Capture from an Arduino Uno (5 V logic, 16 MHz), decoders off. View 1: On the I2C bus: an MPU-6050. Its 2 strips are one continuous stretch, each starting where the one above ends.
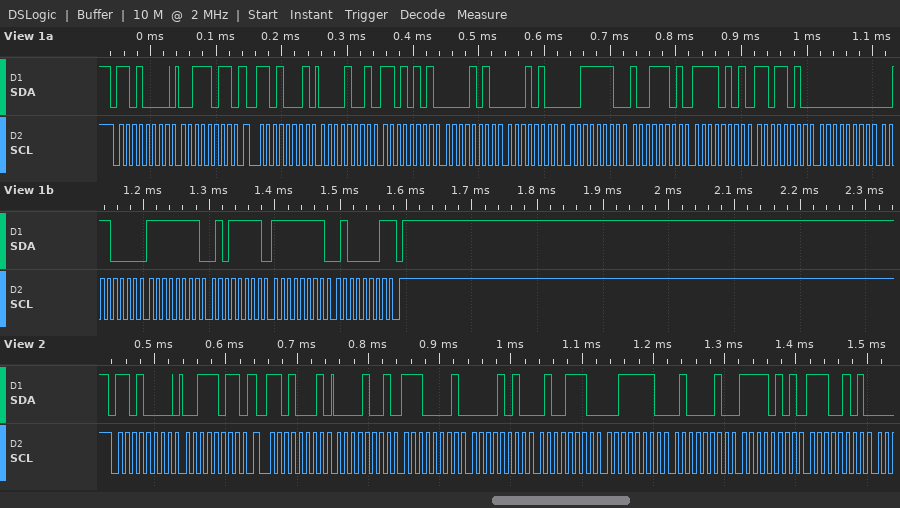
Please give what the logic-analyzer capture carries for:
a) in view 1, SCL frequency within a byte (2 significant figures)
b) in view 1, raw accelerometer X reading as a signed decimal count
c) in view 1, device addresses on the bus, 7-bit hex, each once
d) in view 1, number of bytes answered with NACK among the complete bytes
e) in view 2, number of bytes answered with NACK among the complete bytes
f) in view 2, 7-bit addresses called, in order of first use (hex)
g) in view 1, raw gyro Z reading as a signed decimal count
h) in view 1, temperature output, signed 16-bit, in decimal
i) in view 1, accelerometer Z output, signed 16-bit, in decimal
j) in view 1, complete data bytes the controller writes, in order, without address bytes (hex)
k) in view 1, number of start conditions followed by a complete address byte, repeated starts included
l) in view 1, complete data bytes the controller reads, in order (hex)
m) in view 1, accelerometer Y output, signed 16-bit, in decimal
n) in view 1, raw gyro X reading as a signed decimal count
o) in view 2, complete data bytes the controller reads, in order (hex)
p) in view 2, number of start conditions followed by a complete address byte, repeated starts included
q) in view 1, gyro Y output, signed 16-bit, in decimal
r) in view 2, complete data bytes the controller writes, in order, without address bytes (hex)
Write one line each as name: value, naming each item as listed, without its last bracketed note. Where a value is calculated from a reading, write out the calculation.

in view 1, SCL frequency within a byte: 100 kHz
in view 1, raw accelerometer X reading as a signed decimal count: 0x09D5 = 2517
in view 1, device addresses on the bus, 7-bit hex, each once: 0x68
in view 1, number of bytes answered with NACK among the complete bytes: 1
in view 2, number of bytes answered with NACK among the complete bytes: 0
in view 2, 7-bit addresses called, in order of first use: 0x68
in view 1, raw gyro Z reading as a signed decimal count: 0xFF41 = -191
in view 1, temperature output, signed 16-bit, in decimal: 0xF5DA = -2598
in view 1, accelerometer Z output, signed 16-bit, in decimal: 0x3E9D = 16029
in view 1, complete data bytes the controller writes, in order, without address bytes: 3B
in view 1, number of start conditions followed by a complete address byte, repeated starts included: 2
in view 1, complete data bytes the controller reads, in order: 09 D5 0A 14 3E 9D F5 DA 00 30 FF 5F FF 41
in view 1, accelerometer Y output, signed 16-bit, in decimal: 0x0A14 = 2580
in view 1, raw gyro X reading as a signed decimal count: 0x0030 = 48
in view 2, complete data bytes the controller reads, in order: 09 E1 0A 4E 3E 42 F5 E5
in view 2, number of start conditions followed by a complete address byte, repeated starts included: 2
in view 1, gyro Y output, signed 16-bit, in decimal: 0xFF5F = -161
in view 2, complete data bytes the controller writes, in order, without address bytes: 3B
